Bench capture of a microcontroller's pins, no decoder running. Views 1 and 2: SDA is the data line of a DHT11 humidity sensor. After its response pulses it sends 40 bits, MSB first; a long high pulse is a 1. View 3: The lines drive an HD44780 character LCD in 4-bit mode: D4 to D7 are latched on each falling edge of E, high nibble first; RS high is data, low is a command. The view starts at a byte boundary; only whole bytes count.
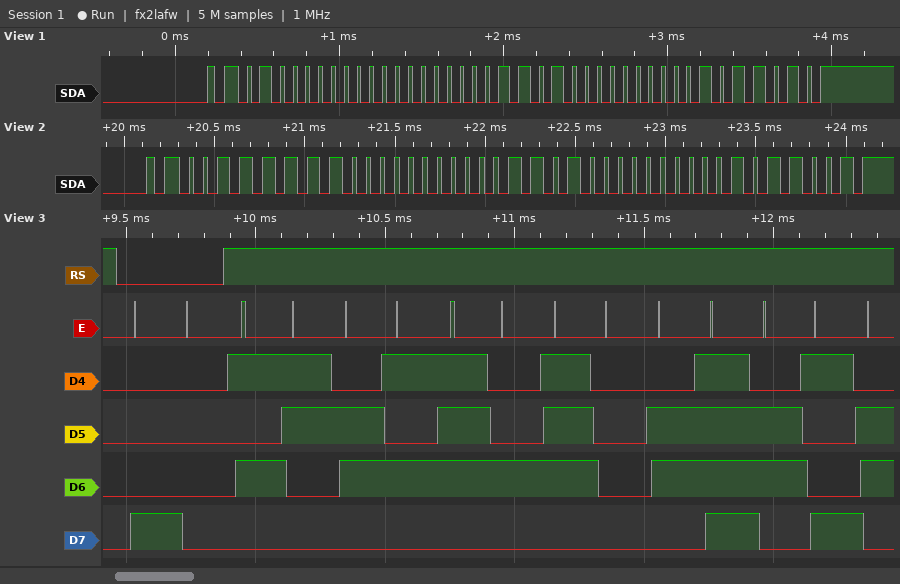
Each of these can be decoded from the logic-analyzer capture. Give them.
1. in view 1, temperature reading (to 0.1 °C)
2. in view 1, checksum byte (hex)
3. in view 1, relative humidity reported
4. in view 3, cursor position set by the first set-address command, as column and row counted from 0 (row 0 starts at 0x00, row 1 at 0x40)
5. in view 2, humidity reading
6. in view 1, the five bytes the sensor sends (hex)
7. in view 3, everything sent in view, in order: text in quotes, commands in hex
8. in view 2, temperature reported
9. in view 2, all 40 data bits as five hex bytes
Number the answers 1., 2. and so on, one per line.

1. 26.0 °C
2. 0x5A
3. 64 %
4. column 0, row 0
5. 63 %
6. 40 00 1A 00 5A
7. 0x80 "Setpoi"
8. 26.0 °C
9. 3F 00 1A 00 59
